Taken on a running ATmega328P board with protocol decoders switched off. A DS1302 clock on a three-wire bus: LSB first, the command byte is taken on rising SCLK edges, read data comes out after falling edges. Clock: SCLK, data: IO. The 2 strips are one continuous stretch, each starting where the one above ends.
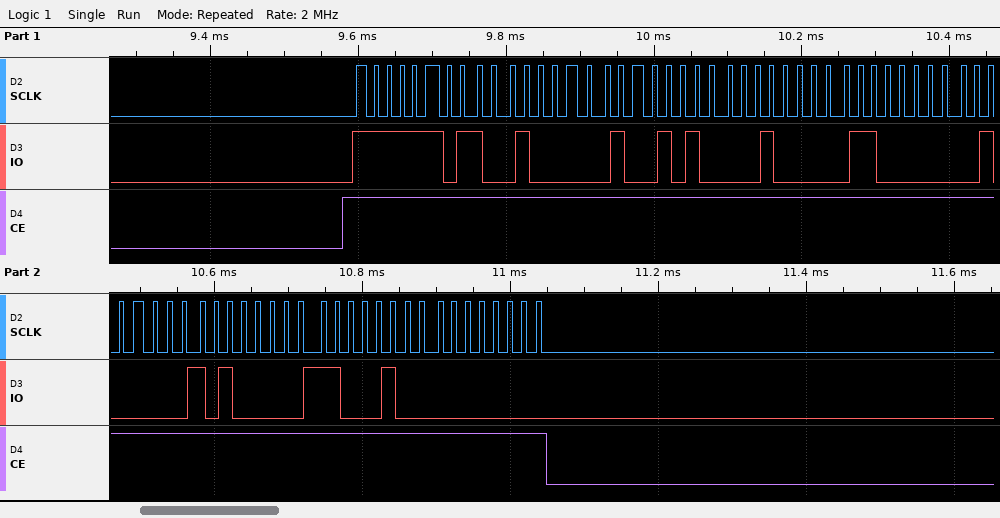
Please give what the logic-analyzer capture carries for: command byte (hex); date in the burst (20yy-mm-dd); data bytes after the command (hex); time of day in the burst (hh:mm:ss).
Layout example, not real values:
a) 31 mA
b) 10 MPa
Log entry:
a) 0xBF
b) 2023-04-06
c) 09 52 08 06 04 05 23 00
d) 08:52:09
